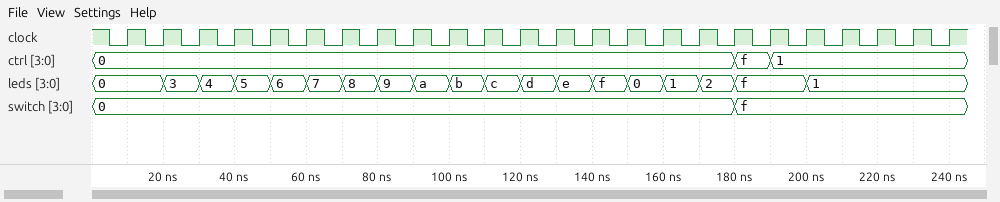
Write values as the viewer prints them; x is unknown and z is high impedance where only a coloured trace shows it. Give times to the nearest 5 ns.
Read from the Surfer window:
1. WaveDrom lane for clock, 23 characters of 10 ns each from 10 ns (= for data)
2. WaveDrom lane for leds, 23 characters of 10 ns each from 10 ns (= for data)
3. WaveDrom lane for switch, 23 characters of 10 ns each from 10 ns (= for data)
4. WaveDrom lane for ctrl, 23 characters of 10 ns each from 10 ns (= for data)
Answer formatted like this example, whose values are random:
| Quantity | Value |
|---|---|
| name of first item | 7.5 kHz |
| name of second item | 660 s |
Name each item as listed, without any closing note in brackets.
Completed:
| Quantity | Value |
|---|---|
| WaveDrom lane for clock, 23 characters of 10 ns each from 10 ns | {name: 'clock', wave: 'p......................'} |
| WaveDrom lane for leds, 23 characters of 10 ns each from 10 ns | {name: 'leds', wave: '==================.=...', data: '0 3 4 5 6 7 8 9 a b c d e f 0 1 2 f 1'} |
| WaveDrom lane for switch, 23 characters of 10 ns each from 10 ns | {name: 'switch', wave: '=................=.....', data: '0 f'} |
| WaveDrom lane for ctrl, 23 characters of 10 ns each from 10 ns | {name: 'ctrl', wave: '=................==....', data: '0 f 1'} |
